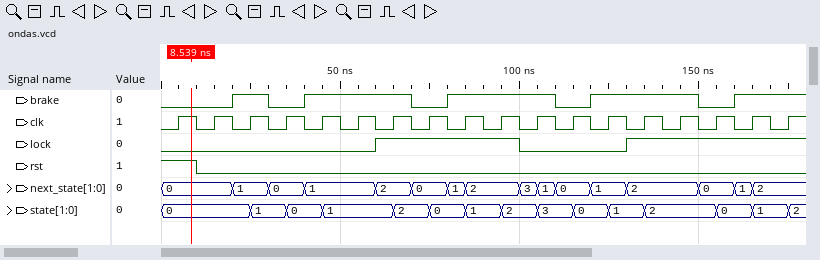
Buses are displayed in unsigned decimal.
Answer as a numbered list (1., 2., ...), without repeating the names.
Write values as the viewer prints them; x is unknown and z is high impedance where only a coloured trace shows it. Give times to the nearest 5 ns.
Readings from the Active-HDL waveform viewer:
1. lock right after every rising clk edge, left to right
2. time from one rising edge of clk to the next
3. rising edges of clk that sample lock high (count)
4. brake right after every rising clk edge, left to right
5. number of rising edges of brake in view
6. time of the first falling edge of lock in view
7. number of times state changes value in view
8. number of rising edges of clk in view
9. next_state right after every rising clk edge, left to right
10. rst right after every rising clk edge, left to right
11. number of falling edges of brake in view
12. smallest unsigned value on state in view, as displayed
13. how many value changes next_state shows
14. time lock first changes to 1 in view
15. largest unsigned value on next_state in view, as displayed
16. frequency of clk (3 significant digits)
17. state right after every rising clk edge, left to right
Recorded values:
1. 0 0 0 0 0 0 1 1 1 1 0 0 0 1 1 1 1 1
2. 10 ns
3. 9
4. 0 0 1 0 1 1 1 0 1 1 1 0 1 1 1 0 1 1
5. 5
6. 100 ns
7. 14
8. 18
9. 0, 0, 1, 0, 1, 1, 2, 0, 2, 2, 1, 0, 1, 2, 2, 0, 2, 2
10. 1 0 0 0 0 0 0 0 0 0 0 0 0 0 0 0 0 0
11. 4
12. 0
13. 15
14. 60 ns
15. 3
16. 100 MHz
17. 0, 0, 1, 0, 1, 1, 2, 0, 1, 2, 3, 0, 1, 2, 2, 0, 1, 2
